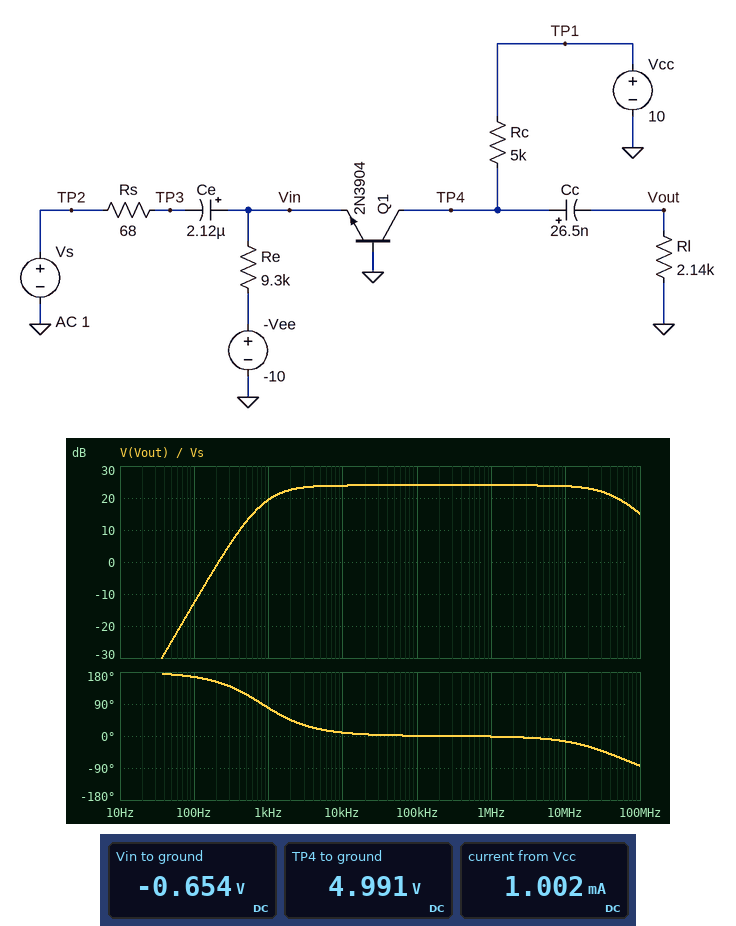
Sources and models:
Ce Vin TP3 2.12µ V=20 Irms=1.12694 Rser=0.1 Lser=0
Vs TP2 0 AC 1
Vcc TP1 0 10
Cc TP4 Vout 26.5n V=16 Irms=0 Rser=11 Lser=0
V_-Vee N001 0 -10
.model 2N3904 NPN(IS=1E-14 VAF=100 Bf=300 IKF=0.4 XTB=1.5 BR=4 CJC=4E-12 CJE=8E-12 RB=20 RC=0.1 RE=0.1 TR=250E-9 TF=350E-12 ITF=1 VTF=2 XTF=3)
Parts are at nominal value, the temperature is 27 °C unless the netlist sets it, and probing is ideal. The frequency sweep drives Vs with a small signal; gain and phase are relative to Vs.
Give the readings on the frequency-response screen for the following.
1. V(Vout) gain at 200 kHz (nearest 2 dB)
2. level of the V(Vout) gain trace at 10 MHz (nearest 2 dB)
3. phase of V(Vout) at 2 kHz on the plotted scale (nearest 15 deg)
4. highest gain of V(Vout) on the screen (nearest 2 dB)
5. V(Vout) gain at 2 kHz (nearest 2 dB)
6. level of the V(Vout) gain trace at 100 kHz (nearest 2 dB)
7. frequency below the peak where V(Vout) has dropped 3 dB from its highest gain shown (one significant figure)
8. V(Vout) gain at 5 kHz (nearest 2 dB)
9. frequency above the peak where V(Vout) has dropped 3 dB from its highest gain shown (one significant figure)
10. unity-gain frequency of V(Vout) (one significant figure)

24 dB
24 dB
45 deg
24 dB
22 dB
24 dB
1 kHz
24 dB
40 MHz
200 Hz
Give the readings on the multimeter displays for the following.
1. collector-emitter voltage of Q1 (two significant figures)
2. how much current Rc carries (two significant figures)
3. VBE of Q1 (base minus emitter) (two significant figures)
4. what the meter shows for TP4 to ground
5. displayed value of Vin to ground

5.6 V
1.0 mA
650 mV
4.991 V
-0.654 V
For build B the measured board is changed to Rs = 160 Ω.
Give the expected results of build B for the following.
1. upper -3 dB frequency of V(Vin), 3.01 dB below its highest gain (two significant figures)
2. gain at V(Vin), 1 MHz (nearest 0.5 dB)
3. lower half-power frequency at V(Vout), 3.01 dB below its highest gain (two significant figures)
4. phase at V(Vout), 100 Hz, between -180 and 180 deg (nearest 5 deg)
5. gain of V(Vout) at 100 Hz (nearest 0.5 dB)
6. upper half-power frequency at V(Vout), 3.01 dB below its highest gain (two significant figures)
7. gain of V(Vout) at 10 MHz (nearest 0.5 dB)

510 MHz
-17.0 dB
1.0 kHz
160 deg
-13.0 dB
44 MHz
18.0 dB
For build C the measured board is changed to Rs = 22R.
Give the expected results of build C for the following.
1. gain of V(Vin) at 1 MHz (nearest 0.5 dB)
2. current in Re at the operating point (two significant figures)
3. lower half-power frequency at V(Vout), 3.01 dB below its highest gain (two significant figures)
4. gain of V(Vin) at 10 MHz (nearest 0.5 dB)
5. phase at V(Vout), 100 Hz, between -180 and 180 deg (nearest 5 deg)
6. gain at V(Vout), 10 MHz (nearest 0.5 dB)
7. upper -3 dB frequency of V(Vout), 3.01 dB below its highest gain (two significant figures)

-5.5 dB
1.0 mA
1.9 kHz
-5.0 dB
170 deg
29.5 dB
35 MHz
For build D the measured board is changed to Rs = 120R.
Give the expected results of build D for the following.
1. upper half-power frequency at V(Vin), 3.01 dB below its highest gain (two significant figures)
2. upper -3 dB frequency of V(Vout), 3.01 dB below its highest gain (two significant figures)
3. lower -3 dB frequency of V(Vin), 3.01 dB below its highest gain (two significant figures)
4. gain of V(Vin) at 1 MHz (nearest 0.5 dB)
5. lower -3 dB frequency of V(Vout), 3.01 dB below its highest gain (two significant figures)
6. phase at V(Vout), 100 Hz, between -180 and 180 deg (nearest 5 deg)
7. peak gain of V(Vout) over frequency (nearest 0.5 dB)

550 MHz
43 MHz
3.0 MHz
-15.0 dB
1.1 kHz
160 deg
20.0 dB
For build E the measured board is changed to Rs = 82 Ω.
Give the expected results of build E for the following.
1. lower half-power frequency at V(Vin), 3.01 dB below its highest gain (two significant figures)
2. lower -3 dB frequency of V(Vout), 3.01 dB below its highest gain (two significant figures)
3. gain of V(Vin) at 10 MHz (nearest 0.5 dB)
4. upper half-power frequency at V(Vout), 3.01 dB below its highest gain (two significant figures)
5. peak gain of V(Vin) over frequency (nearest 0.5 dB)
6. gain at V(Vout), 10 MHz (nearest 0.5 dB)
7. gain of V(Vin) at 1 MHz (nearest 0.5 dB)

2.8 kHz
1.2 kHz
-12.0 dB
41 MHz
-9.5 dB
22.5 dB
-12.5 dB
